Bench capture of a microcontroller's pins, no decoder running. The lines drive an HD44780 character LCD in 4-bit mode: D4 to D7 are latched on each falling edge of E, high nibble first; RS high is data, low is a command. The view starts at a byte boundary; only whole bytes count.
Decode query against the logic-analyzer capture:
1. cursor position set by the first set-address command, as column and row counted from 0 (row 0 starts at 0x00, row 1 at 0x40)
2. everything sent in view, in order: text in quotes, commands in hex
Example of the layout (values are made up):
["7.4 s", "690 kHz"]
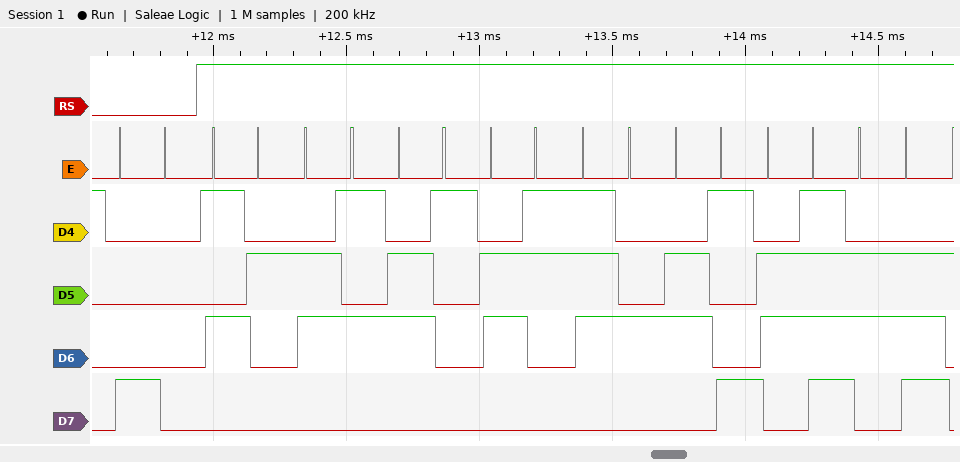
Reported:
["column 0, row 0", "0x80 \"Reaction\""]
